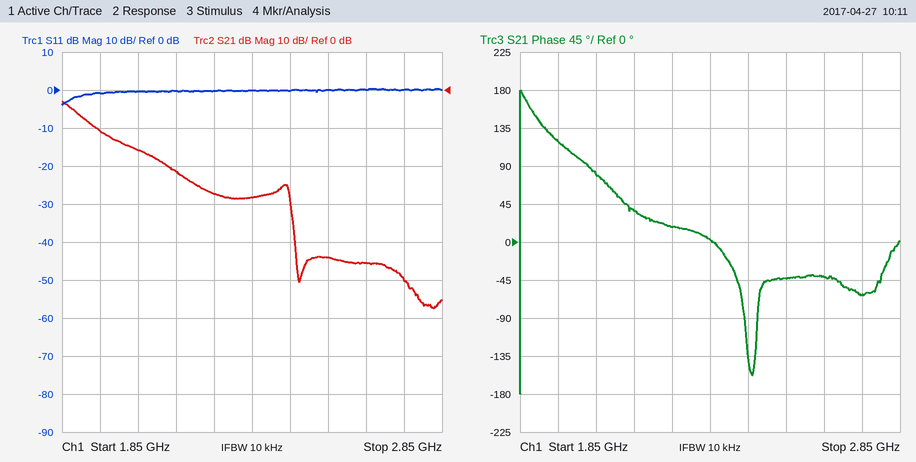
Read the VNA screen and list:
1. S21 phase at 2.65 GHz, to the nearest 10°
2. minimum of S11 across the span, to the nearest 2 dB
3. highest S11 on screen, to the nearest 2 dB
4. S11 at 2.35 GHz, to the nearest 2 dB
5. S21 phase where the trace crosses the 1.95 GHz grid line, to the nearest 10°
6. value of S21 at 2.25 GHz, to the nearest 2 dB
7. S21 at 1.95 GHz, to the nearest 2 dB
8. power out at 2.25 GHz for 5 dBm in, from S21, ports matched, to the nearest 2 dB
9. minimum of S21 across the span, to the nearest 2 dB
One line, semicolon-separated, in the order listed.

-40°; -4 dB; 0 dB; 0 dB; 120°; -28 dB; -10 dB; -22 dBm; -58 dB
